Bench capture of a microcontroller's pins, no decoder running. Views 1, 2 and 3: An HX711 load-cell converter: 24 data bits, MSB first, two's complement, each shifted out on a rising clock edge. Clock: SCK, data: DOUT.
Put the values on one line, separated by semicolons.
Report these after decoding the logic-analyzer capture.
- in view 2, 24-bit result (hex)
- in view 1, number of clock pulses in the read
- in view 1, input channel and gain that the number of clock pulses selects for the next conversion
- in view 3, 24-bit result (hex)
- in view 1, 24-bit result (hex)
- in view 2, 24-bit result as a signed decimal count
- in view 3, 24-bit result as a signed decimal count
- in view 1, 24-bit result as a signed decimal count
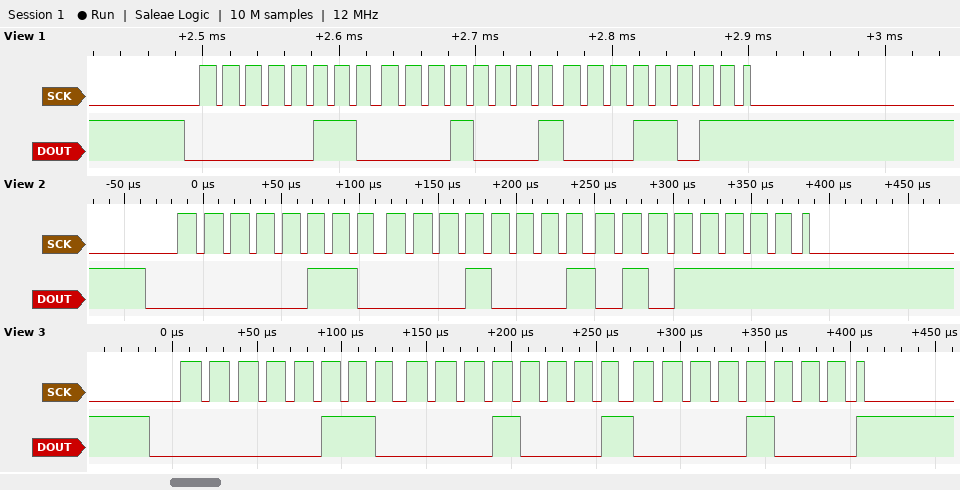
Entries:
0x06115F; 25; channel A, gain 128; 0x061108; 0x06111B; 397663; 397576; 397595
